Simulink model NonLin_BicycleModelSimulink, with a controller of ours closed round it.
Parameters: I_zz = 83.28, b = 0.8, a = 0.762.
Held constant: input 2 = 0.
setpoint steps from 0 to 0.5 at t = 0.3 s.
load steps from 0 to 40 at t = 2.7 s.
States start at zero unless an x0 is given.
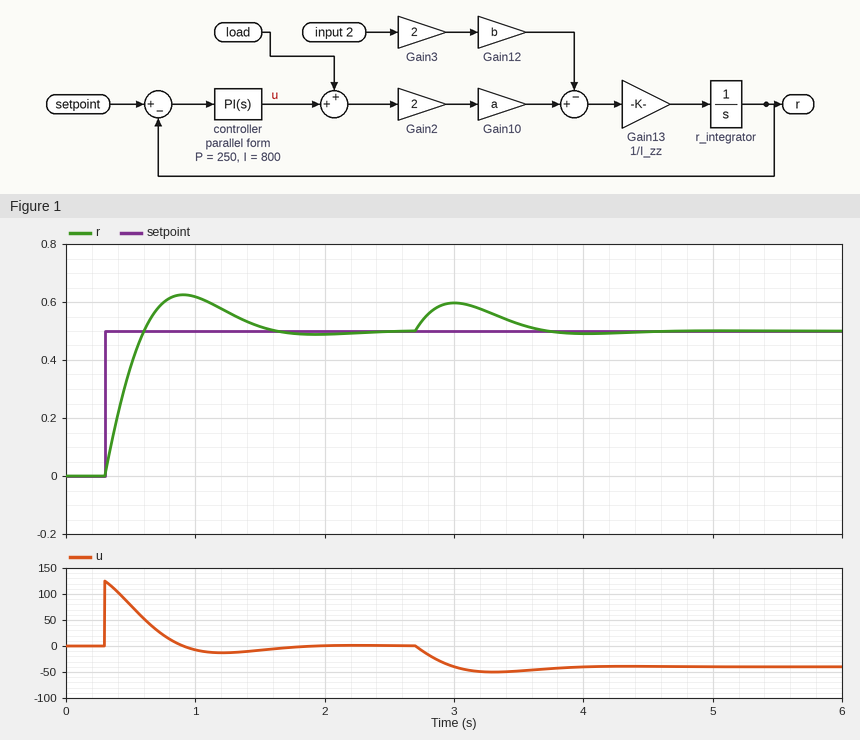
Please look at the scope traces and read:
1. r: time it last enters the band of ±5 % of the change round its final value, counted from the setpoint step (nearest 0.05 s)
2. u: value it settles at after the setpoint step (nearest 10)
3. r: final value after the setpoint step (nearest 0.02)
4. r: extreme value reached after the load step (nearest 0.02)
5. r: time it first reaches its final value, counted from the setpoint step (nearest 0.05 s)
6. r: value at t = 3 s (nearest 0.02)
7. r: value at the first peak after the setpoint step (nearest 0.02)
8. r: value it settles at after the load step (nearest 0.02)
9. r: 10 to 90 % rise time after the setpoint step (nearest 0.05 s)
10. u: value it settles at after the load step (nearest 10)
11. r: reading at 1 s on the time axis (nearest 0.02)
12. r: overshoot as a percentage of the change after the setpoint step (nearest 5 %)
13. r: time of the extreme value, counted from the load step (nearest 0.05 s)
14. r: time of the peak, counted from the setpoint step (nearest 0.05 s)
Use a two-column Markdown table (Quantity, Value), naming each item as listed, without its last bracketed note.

| Quantity | Value |
|---|---|
| r: time it last enters the band of ±5 % of the change round its final value, counted from the setpoint step | 1.15 s |
| u: value it settles at after the setpoint step | 0 |
| r: final value after the setpoint step | 0.50 |
| r: extreme value reached after the load step | 0.60 |
| r: time it first reaches its final value, counted from the setpoint step | 0.30 s |
| r: value at t = 3 s | 0.60 |
| r: value at the first peak after the setpoint step | 0.62 |
| r: value it settles at after the load step | 0.50 |
| r: 10 to 90 % rise time after the setpoint step | 0.25 s |
| u: value it settles at after the load step | -40 |
| r: reading at 1 s on the time axis | 0.62 |
| r: overshoot as a percentage of the change after the setpoint step | 25 % |
| r: time of the extreme value, counted from the load step | 0.30 s |
| r: time of the peak, counted from the setpoint step | 0.60 s |
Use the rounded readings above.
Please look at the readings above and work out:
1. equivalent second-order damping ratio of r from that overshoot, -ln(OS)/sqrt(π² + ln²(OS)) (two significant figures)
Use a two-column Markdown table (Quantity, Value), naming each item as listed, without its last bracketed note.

| Quantity | Value |
|---|---|
| equivalent second-order damping ratio of r from that overshoot, -ln(OS)/sqrt(π² + ln²(OS)) | 0.40 |
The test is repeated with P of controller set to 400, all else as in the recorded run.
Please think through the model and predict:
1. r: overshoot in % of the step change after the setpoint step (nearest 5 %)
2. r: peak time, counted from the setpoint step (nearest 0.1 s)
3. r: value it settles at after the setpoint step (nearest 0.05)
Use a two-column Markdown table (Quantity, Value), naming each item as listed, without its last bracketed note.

| Quantity | Value |
|---|---|
| r: overshoot in % of the step change after the setpoint step | 15 % |
| r: peak time, counted from the setpoint step | 0.5 s |
| r: value it settles at after the setpoint step | 0.50 |
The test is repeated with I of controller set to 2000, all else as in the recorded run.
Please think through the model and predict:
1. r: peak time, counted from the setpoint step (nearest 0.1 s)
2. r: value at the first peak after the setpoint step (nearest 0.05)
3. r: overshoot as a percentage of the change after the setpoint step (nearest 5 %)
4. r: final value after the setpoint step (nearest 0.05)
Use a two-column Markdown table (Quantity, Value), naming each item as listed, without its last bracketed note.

| Quantity | Value |
|---|---|
| r: peak time, counted from the setpoint step | 0.4 s |
| r: value at the first peak after the setpoint step | 0.70 |
| r: overshoot as a percentage of the change after the setpoint step | 40 % |
| r: final value after the setpoint step | 0.50 |
